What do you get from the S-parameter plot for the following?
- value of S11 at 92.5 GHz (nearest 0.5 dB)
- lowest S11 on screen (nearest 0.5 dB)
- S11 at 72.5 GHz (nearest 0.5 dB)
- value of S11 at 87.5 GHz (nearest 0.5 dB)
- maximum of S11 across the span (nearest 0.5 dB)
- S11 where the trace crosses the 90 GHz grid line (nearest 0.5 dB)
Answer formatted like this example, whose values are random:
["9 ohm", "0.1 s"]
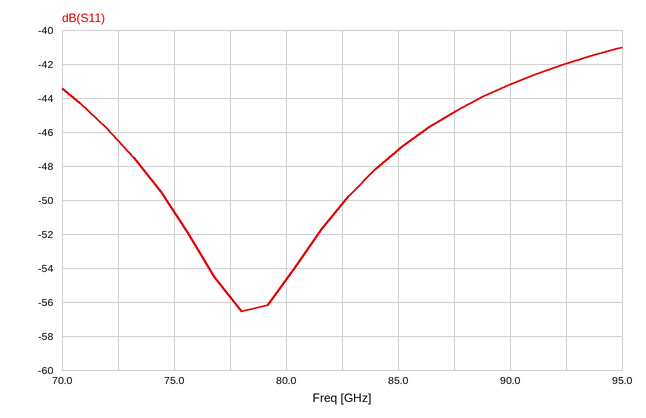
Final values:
["-42.0 dB", "-56.5 dB", "-46.5 dB", "-45.0 dB", "-41.0 dB", "-43.0 dB"]
